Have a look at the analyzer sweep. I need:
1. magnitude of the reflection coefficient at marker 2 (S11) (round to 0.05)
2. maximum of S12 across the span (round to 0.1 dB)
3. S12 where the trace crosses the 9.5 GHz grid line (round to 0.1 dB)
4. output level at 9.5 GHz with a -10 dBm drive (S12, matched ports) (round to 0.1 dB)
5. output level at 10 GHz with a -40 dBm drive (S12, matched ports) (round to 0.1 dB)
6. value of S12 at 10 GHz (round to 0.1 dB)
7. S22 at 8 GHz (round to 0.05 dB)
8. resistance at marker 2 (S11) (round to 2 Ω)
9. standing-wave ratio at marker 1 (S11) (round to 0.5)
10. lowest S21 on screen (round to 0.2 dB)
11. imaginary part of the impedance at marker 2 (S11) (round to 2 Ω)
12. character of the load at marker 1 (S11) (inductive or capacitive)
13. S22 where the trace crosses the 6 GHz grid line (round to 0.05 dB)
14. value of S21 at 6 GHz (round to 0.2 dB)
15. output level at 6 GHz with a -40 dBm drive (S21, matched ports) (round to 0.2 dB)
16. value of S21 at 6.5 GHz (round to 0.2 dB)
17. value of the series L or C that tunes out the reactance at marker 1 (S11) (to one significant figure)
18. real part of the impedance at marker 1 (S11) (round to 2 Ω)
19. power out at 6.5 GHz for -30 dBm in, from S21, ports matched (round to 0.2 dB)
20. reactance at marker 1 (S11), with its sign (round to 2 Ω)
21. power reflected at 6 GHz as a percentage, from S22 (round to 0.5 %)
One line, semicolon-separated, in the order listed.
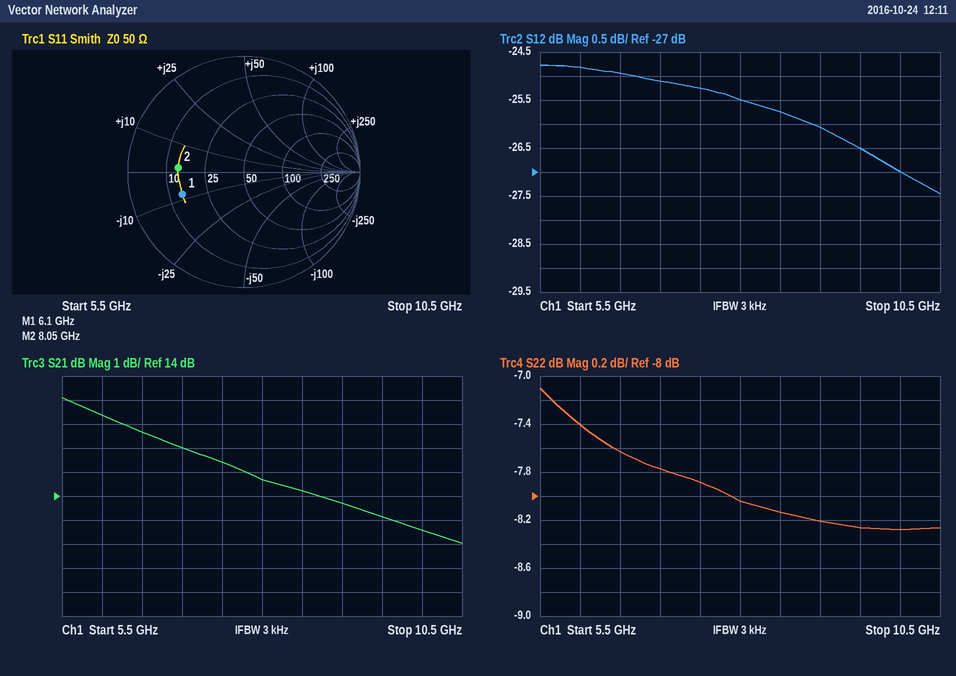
0.55; -24.8 dB; -26.5 dB; -36.5 dBm; -67.0 dBm; -27.0 dB; -8.05 dB; 14 Ω; 3.5; 12.0 dB; +2 Ω; capacitive; -7.40 dB; 17.4 dB; -22.6 dBm; 16.6 dB; 200 pH; 14 Ω; -13.4 dBm; -8 Ω; 18.0 %
